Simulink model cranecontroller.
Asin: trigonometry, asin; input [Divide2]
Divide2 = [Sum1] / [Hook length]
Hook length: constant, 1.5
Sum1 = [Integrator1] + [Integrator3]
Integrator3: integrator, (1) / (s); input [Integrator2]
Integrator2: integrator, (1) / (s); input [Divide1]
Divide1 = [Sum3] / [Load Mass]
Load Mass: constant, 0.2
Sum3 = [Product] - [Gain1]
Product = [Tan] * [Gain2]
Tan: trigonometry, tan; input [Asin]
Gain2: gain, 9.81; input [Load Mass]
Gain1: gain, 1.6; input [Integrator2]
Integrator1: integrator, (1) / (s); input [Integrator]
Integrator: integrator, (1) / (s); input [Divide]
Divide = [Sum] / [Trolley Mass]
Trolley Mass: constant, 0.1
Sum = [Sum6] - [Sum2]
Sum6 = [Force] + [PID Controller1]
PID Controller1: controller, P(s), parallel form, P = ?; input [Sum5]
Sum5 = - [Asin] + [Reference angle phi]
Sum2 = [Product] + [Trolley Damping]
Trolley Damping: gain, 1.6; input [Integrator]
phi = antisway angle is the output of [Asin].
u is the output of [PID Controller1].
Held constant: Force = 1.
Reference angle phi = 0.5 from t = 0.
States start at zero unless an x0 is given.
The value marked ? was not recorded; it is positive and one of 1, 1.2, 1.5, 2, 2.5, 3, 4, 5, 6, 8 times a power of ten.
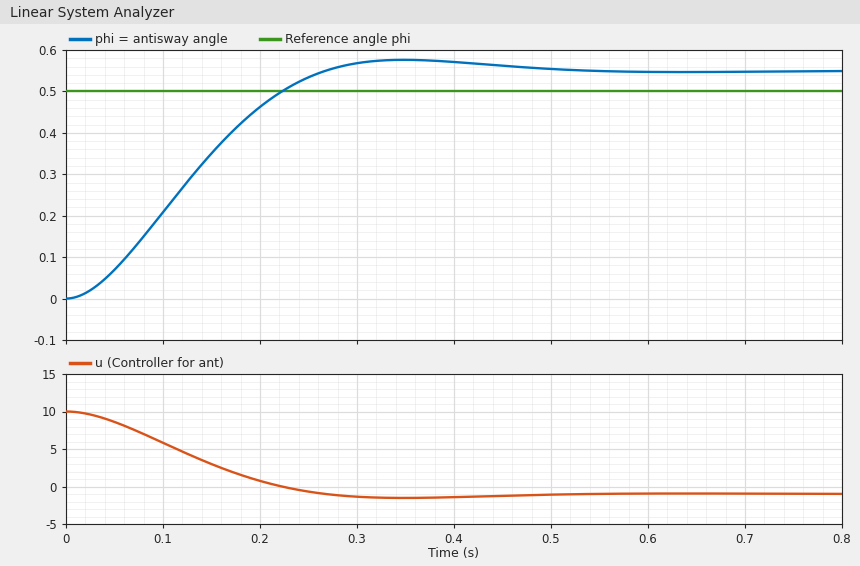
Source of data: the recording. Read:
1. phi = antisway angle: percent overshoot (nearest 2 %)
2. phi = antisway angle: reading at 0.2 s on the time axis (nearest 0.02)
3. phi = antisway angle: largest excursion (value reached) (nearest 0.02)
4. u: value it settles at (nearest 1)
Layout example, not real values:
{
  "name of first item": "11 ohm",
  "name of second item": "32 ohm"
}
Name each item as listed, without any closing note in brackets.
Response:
{
  "phi = antisway angle: percent overshoot": "4 %",
  "phi = antisway angle: reading at 0.2 s on the time axis": "0.46",
  "phi = antisway angle: largest excursion (value reached)": "0.58",
  "u: value it settles at": "-1"
}
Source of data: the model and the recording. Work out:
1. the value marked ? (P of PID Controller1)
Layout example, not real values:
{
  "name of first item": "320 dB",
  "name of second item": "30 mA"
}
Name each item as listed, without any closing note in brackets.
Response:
{
  "the value marked ?": "20"
}
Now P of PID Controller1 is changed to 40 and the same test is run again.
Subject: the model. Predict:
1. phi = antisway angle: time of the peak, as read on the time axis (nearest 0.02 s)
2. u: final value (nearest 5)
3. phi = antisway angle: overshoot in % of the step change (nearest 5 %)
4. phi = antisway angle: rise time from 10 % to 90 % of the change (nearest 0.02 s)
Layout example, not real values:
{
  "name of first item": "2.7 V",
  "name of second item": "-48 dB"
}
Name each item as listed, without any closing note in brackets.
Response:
{
  "phi = antisway angle: time of the peak, as read on the time axis": "0.20 s",
  "u: final value": "0",
  "phi = antisway angle: overshoot in % of the step change": "20 %",
  "phi = antisway angle: rise time from 10 % to 90 % of the change": "0.10 s"
}
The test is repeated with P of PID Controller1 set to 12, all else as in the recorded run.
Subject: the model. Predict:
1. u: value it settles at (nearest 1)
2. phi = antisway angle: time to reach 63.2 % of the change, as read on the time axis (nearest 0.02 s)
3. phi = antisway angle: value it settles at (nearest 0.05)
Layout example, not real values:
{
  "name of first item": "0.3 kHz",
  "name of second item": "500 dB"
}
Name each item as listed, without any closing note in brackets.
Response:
{
  "u: value it settles at": "-1",
  "phi = antisway angle: time to reach 63.2 % of the change, as read on the time axis": "0.22 s",
  "phi = antisway angle: value it settles at": "0.60"
}
